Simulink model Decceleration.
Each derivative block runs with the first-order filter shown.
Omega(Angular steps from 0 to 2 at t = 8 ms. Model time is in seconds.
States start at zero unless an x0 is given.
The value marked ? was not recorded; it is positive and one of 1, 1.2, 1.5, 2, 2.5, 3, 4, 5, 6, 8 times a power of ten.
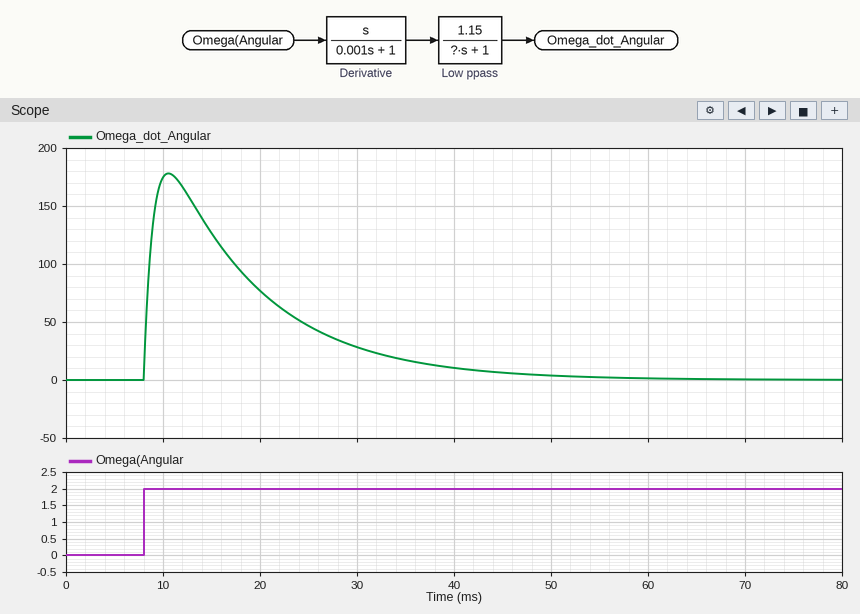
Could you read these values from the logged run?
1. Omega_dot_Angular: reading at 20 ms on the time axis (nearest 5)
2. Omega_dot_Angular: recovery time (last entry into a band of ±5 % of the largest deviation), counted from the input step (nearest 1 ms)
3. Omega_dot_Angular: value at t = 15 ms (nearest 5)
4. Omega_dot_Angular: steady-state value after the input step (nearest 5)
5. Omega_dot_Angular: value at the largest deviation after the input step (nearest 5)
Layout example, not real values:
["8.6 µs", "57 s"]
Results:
["75", "34 ms", "125", "0", "180"]
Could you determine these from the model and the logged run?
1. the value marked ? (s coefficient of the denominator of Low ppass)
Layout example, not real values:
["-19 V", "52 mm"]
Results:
["0.01"]
